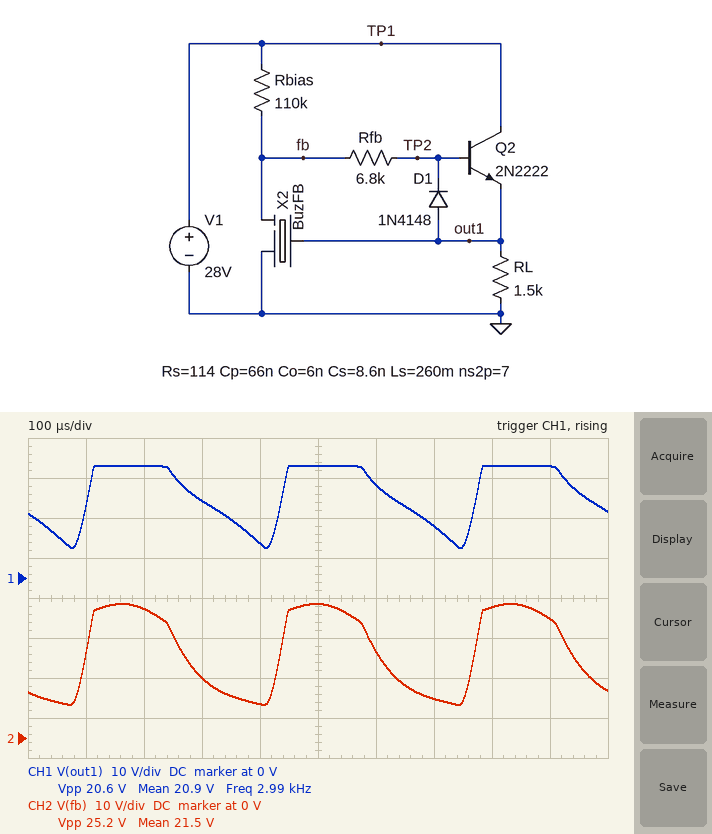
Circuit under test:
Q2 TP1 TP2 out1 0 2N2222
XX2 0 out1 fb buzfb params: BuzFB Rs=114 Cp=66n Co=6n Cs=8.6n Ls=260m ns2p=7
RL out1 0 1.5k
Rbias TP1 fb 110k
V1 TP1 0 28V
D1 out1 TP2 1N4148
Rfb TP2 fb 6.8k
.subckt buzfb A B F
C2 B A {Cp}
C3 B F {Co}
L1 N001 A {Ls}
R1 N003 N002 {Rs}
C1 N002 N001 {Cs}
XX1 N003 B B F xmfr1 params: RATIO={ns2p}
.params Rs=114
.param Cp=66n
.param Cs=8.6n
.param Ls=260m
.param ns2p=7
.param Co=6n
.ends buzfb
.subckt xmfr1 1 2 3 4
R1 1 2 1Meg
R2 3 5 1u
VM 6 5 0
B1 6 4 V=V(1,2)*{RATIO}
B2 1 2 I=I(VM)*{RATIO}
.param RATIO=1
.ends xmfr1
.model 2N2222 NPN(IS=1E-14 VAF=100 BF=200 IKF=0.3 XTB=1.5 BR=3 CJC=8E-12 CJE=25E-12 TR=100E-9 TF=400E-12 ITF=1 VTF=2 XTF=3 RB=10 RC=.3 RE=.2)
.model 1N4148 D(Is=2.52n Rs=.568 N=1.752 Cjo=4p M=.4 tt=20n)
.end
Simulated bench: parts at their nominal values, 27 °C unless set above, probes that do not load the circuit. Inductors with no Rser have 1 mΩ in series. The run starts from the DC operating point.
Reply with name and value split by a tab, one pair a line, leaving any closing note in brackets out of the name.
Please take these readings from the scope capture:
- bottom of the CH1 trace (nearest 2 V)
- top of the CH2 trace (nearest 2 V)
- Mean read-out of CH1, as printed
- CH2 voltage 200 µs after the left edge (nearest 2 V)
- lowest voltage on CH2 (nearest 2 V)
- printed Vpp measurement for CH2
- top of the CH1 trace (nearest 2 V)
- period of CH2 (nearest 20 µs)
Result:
bottom of the CH1 trace	8 V
top of the CH2 trace	34 V
Mean read-out of CH1, as printed	20.9 V
CH2 voltage 200 µs after the left edge	32 V
lowest voltage on CH2	8 V
printed Vpp measurement for CH2	25.2 V
top of the CH1 trace	28 V
period of CH2	340 µs
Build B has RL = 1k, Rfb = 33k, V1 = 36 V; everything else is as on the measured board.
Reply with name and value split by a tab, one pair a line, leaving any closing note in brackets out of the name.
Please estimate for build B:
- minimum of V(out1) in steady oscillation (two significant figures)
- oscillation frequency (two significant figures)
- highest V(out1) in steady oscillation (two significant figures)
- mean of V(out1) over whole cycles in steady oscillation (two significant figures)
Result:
minimum of V(out1) in steady oscillation	3.8 V
oscillation frequency	2.1 kHz
highest V(out1) in steady oscillation	36 V
mean of V(out1) over whole cycles in steady oscillation	21 V
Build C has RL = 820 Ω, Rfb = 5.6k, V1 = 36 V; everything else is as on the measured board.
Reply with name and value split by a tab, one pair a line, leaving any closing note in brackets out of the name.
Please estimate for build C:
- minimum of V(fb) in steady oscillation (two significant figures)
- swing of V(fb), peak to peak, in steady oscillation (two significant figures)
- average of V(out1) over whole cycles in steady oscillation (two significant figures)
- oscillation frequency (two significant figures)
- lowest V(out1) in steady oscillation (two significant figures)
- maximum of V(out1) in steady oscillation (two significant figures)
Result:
minimum of V(fb) in steady oscillation	5.4 V
swing of V(fb), peak to peak, in steady oscillation	44 V
average of V(out1) over whole cycles in steady oscillation	26 V
oscillation frequency	3.2 kHz
lowest V(out1) in steady oscillation	5.0 V
maximum of V(out1) in steady oscillation	36 V
